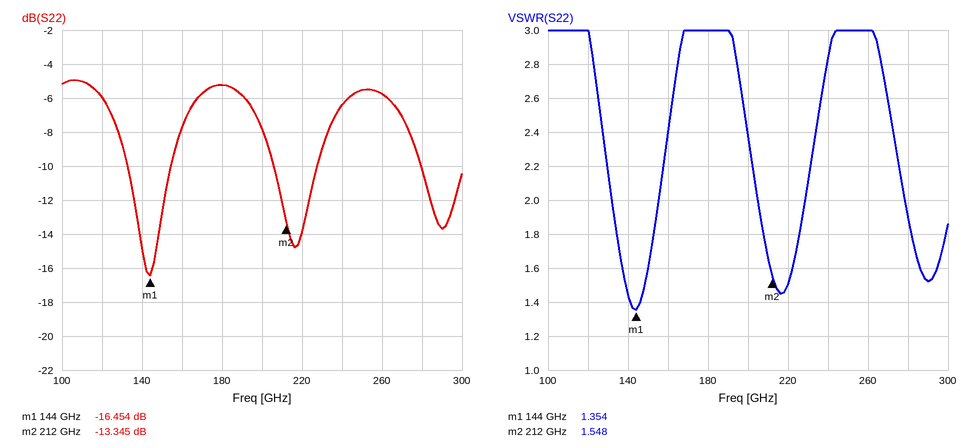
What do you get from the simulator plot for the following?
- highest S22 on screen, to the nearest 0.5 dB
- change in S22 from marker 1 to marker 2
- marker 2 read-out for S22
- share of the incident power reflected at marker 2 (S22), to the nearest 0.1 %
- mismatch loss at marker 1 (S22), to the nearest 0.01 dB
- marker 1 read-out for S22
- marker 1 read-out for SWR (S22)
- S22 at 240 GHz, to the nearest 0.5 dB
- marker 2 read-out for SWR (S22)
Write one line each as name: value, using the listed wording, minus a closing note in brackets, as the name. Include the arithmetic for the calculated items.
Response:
highest S22 on screen, to the nearest 0.5 dB: -5.0 dB
change in S22 from marker 1 to marker 2: -13.345 − (-16.454) = 3.109 dB
marker 2 read-out for S22: -13.345 dB
share of the incident power reflected at marker 2 (S22), to the nearest 0.1 %: 10^(-13.345/10) ≈ 4.6 %
mismatch loss at marker 1 (S22), to the nearest 0.01 dB: −10 log10(1 − 10^(-16.454/10)) ≈ 0.10 dB
marker 1 read-out for S22: -16.454 dB
marker 1 read-out for SWR: 1.354
S22 at 240 GHz, to the nearest 0.5 dB: -6.5 dB
marker 2 read-out for SWR: 1.548
